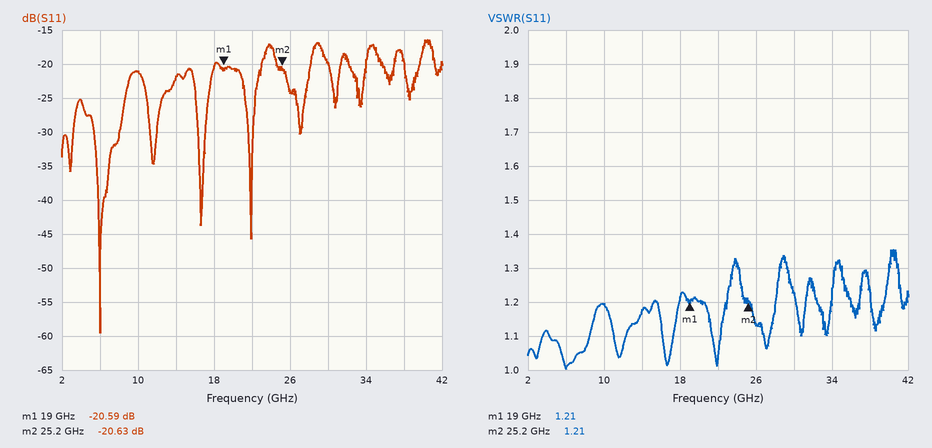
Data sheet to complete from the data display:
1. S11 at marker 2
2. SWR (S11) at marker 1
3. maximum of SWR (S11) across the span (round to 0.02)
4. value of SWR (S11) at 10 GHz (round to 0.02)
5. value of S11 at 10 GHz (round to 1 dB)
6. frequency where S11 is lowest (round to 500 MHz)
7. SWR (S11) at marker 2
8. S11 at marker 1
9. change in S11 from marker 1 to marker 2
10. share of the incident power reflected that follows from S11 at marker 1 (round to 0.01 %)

-20.63 dB
1.21
1.36
1.20
-21 dB
6.0 GHz
1.21
-20.59 dB
-0.04 dB
0.87 %
